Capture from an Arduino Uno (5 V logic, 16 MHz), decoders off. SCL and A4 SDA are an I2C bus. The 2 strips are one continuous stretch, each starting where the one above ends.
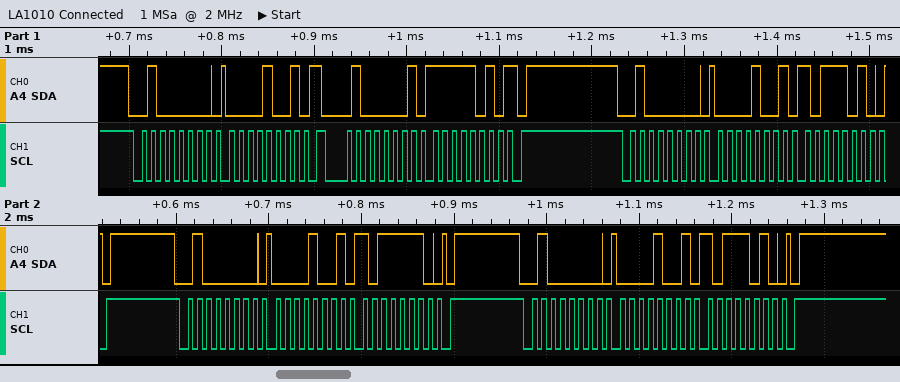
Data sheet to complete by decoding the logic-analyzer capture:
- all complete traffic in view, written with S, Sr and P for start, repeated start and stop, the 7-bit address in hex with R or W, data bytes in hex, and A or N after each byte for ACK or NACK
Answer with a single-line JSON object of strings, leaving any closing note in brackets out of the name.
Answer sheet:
{"all complete traffic in view, written with S, Sr and P for start, repeated start and stop, the 7-bit address in hex with R or W, data bytes in hex, and A or N after each byte for ACK or NACK": "S 20W A 09 A Sr 20R A FA N P S 20W A 09 A BA A P S 20W A 09 A BE A P S 20W A 09 A BA A P"}
